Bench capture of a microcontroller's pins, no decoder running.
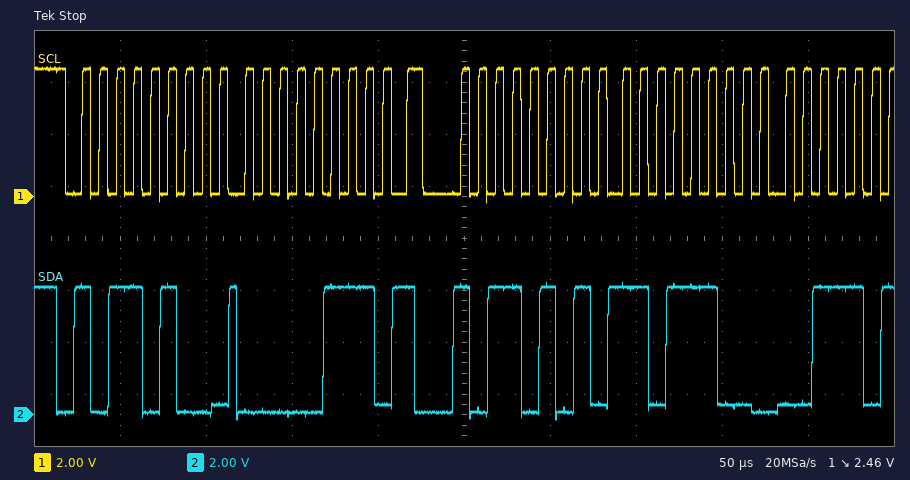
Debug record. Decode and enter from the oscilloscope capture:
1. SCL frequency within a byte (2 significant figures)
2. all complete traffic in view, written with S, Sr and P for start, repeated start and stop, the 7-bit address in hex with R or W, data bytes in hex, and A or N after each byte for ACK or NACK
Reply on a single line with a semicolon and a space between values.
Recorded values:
100 kHz; S 5AW A 07 A Sr 5AR A DC A
